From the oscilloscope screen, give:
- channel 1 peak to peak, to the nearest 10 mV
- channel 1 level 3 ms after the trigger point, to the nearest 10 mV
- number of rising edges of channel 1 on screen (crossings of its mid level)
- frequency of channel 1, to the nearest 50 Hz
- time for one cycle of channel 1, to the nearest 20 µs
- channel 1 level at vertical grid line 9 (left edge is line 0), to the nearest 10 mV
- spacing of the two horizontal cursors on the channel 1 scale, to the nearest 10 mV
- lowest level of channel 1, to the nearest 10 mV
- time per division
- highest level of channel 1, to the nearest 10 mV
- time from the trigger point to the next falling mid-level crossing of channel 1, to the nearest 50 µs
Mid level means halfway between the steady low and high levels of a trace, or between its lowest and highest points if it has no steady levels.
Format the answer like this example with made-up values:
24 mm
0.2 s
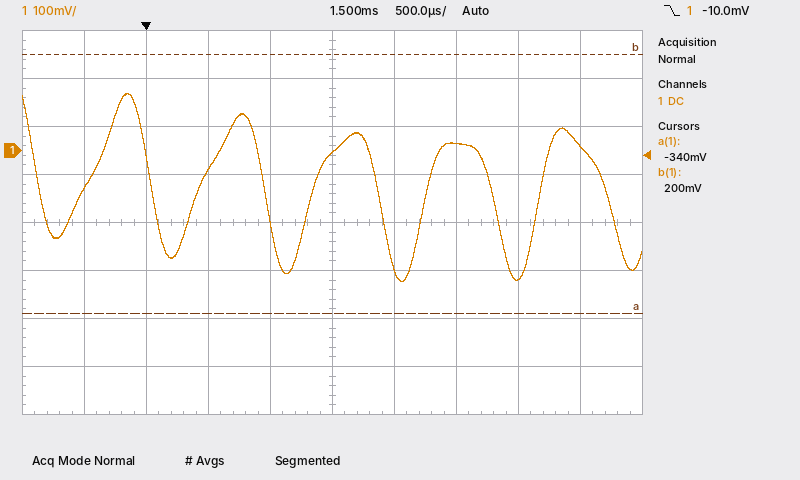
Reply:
390 mV
-270 mV
5
1.10 kHz
920 µs
10 mV
540 mV
-270 mV
500 µs
120 mV
50 µs
